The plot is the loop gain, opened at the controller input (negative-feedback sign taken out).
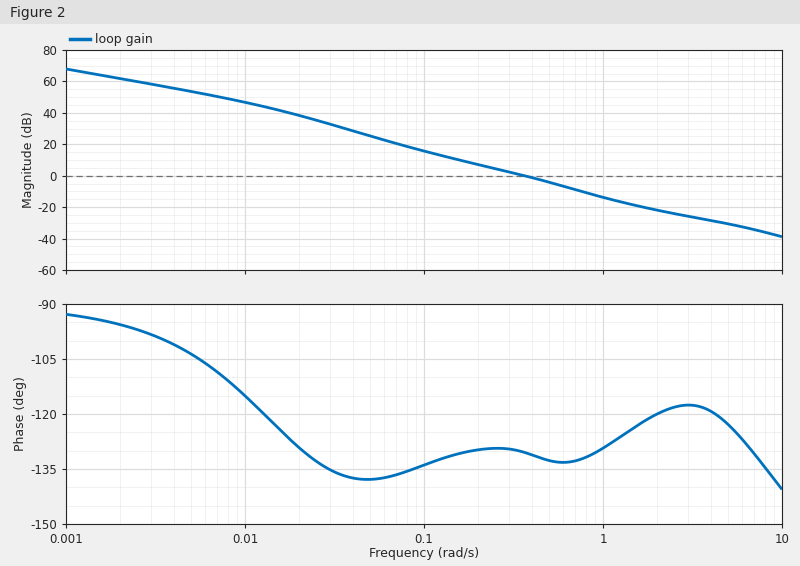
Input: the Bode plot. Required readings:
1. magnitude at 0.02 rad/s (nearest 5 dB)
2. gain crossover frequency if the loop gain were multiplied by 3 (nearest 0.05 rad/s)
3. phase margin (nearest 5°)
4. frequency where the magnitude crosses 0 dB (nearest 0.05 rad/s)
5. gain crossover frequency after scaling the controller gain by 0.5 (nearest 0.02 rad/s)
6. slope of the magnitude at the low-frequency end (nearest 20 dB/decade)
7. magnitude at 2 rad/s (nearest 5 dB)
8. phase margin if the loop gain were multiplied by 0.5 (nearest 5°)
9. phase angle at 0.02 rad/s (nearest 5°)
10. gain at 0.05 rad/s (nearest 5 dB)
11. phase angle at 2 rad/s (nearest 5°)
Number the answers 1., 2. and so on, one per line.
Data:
1. 40 dB
2. 0.75 rad/s
3. 50°
4. 0.35 rad/s
5. 0.22 rad/s
6. -20 dB/decade
7. -20 dB
8. 50°
9. -130°
10. 25 dB
11. -120°
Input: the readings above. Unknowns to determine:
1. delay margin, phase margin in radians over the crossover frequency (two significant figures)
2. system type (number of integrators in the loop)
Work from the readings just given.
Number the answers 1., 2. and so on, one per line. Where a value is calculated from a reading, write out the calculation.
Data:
1. 50 × π / 180 / 0.35 = 2.5 s
2. 1
